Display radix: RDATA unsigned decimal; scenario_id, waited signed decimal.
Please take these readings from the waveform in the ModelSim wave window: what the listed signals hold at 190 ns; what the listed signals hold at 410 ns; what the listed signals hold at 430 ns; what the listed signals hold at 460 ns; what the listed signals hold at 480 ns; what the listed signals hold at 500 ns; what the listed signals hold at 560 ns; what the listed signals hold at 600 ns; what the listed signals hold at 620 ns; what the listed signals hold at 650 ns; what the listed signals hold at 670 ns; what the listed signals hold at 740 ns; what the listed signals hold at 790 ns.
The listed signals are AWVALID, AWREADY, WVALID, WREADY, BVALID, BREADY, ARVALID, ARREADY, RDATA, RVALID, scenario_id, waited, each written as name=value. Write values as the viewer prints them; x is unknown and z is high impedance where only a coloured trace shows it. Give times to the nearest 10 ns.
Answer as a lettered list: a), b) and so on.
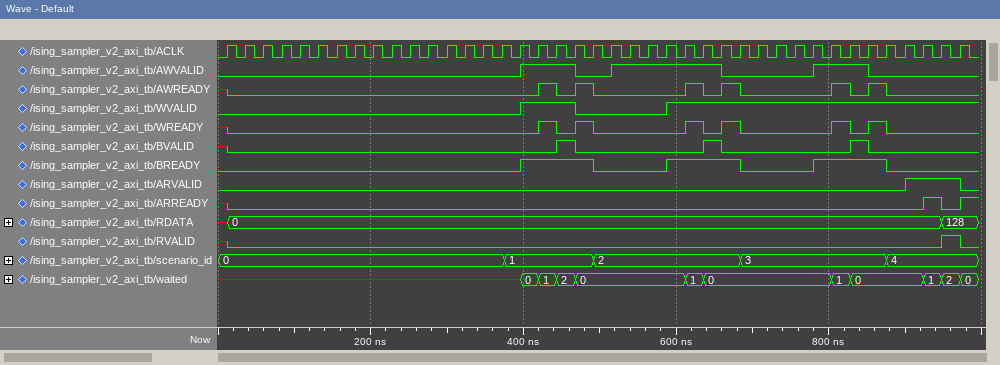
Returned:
a) AWVALID=0, AWREADY=0, WVALID=0, WREADY=0, BVALID=0, BREADY=0, ARVALID=0, ARREADY=0, RDATA=0, RVALID=0, scenario_id=0, waited=x
b) AWVALID=1, AWREADY=0, WVALID=1, WREADY=0, BVALID=0, BREADY=1, ARVALID=0, ARREADY=0, RDATA=0, RVALID=0, scenario_id=1, waited=0
c) AWVALID=1, AWREADY=1, WVALID=1, WREADY=1, BVALID=0, BREADY=1, ARVALID=0, ARREADY=0, RDATA=0, RVALID=0, scenario_id=1, waited=1
d) AWVALID=1, AWREADY=0, WVALID=1, WREADY=0, BVALID=1, BREADY=1, ARVALID=0, ARREADY=0, RDATA=0, RVALID=0, scenario_id=1, waited=2
e) AWVALID=0, AWREADY=1, WVALID=0, WREADY=1, BVALID=0, BREADY=1, ARVALID=0, ARREADY=0, RDATA=0, RVALID=0, scenario_id=1, waited=0
f) AWVALID=0, AWREADY=0, WVALID=0, WREADY=0, BVALID=0, BREADY=0, ARVALID=0, ARREADY=0, RDATA=0, RVALID=0, scenario_id=2, waited=0
g) AWVALID=1, AWREADY=0, WVALID=0, WREADY=0, BVALID=0, BREADY=0, ARVALID=0, ARREADY=0, RDATA=0, RVALID=0, scenario_id=2, waited=0
h) AWVALID=1, AWREADY=0, WVALID=1, WREADY=0, BVALID=0, BREADY=1, ARVALID=0, ARREADY=0, RDATA=0, RVALID=0, scenario_id=2, waited=0
i) AWVALID=1, AWREADY=1, WVALID=1, WREADY=1, BVALID=0, BREADY=1, ARVALID=0, ARREADY=0, RDATA=0, RVALID=0, scenario_id=2, waited=1
j) AWVALID=1, AWREADY=0, WVALID=1, WREADY=0, BVALID=1, BREADY=1, ARVALID=0, ARREADY=0, RDATA=0, RVALID=0, scenario_id=2, waited=0
k) AWVALID=0, AWREADY=1, WVALID=1, WREADY=1, BVALID=0, BREADY=1, ARVALID=0, ARREADY=0, RDATA=0, RVALID=0, scenario_id=2, waited=0
l) AWVALID=0, AWREADY=0, WVALID=1, WREADY=0, BVALID=0, BREADY=0, ARVALID=0, ARREADY=0, RDATA=0, RVALID=0, scenario_id=3, waited=0
m) AWVALID=1, AWREADY=0, WVALID=1, WREADY=0, BVALID=0, BREADY=1, ARVALID=0, ARREADY=0, RDATA=0, RVALID=0, scenario_id=3, waited=0
